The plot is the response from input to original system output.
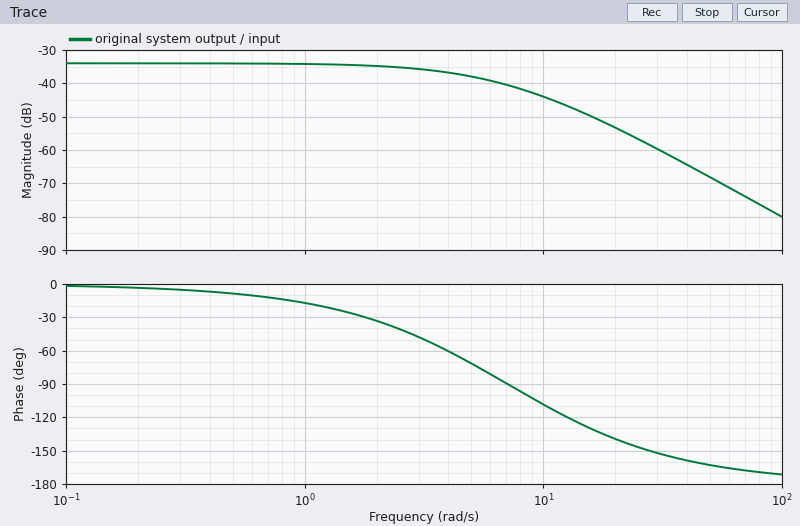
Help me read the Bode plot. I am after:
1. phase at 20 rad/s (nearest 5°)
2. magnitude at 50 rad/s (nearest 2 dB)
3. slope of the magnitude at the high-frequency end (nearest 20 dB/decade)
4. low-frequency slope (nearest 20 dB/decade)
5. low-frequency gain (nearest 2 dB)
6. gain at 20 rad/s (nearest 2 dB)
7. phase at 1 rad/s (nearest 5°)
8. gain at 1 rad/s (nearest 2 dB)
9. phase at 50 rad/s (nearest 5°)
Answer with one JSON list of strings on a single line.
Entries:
["-140°", "-68 dB", "-40 dB/decade", "0 dB/decade", "-34 dB", "-54 dB", "-15°", "-34 dB", "-165°"]
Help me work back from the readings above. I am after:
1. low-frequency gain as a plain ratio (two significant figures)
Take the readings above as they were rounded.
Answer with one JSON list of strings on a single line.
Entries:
["0.020"]
